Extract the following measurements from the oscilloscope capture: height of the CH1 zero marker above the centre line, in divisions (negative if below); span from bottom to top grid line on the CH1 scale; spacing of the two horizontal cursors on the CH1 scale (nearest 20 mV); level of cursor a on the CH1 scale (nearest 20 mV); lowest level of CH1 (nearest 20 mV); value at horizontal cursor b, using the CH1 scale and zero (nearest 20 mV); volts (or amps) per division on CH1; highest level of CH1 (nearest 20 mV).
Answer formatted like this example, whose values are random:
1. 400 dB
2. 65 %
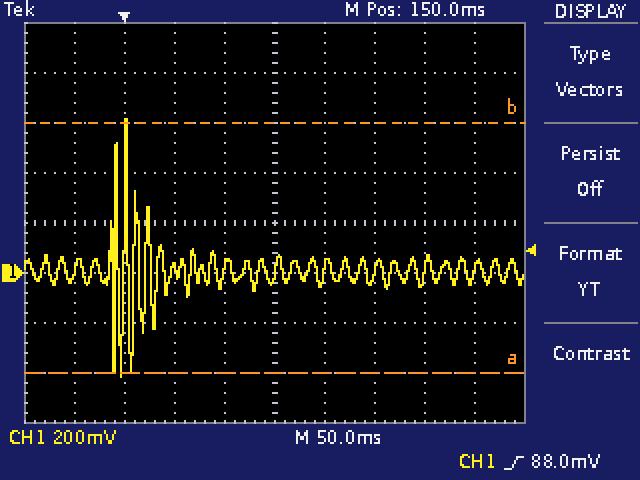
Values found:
1. -1.0 div
2. 1.6 V
3. 1.00 V
4. -400 mV
5. -420 mV
6. 600 mV
7. 200 mV
8. 620 mV
